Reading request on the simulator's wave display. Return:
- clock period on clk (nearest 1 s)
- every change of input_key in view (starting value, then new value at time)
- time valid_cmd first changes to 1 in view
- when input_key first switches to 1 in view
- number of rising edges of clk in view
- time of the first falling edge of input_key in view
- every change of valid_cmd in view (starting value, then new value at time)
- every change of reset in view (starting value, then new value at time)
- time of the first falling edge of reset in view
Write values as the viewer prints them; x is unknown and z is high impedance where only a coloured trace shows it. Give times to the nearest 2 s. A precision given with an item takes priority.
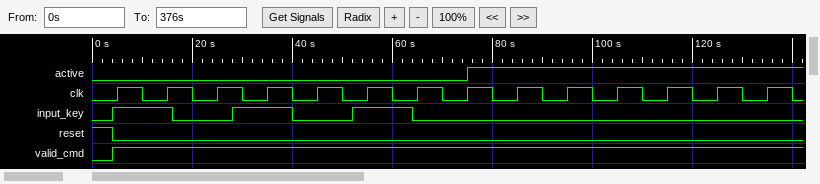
10 s
0, 1 at 4 s, 0 at 16 s, 1 at 28 s, 0 at 40 s, 1 at 52 s, 0 at 64 s
4 s
4 s
14
16 s
0, 1 at 4 s
1, 0 at 4 s
4 s
